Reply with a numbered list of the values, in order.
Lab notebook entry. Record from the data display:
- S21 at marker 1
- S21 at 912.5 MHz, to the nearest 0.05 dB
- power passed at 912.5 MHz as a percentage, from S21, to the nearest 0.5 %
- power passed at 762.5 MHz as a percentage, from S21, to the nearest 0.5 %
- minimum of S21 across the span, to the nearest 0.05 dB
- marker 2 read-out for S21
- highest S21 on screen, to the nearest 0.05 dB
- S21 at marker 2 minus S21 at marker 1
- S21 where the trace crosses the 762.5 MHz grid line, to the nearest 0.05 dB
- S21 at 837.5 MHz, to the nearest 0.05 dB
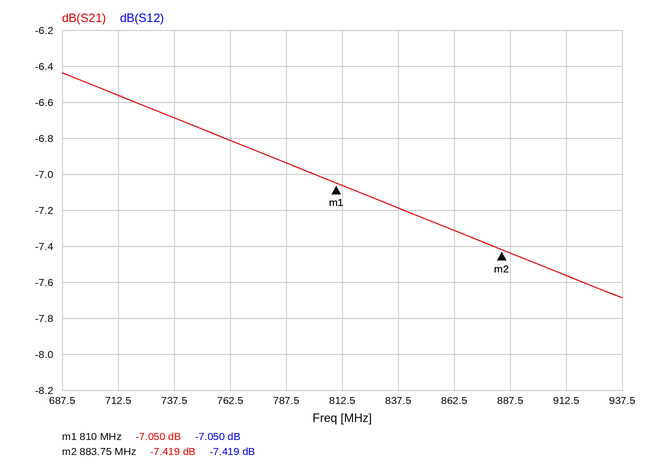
1. -7.050 dB
2. -7.55 dB
3. 17.5 %
4. 21.0 %
5. -7.70 dB
6. -7.419 dB
7. -6.45 dB
8. -0.369 dB
9. -6.80 dB
10. -7.20 dB
